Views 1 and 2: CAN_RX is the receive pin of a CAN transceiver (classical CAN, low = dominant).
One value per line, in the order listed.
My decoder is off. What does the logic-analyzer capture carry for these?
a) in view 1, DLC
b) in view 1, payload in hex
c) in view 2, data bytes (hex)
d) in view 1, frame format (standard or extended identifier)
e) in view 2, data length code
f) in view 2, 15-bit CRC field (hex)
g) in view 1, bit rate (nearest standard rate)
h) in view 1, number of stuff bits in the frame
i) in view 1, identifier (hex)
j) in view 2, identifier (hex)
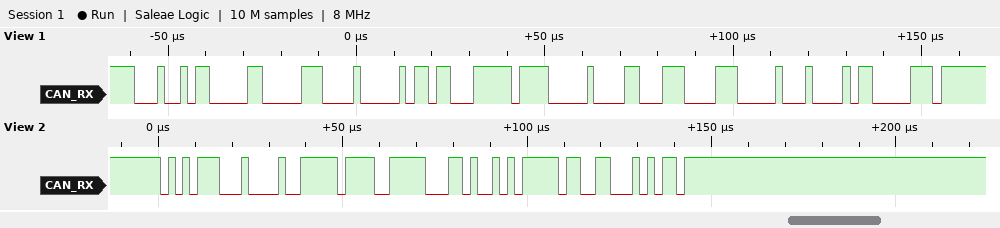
8
30 81 B1 FF 00 63 87 00
FF 9F 34 AF
standard
4
0x7315
500 kbit/s
7
0x12C
0x571
